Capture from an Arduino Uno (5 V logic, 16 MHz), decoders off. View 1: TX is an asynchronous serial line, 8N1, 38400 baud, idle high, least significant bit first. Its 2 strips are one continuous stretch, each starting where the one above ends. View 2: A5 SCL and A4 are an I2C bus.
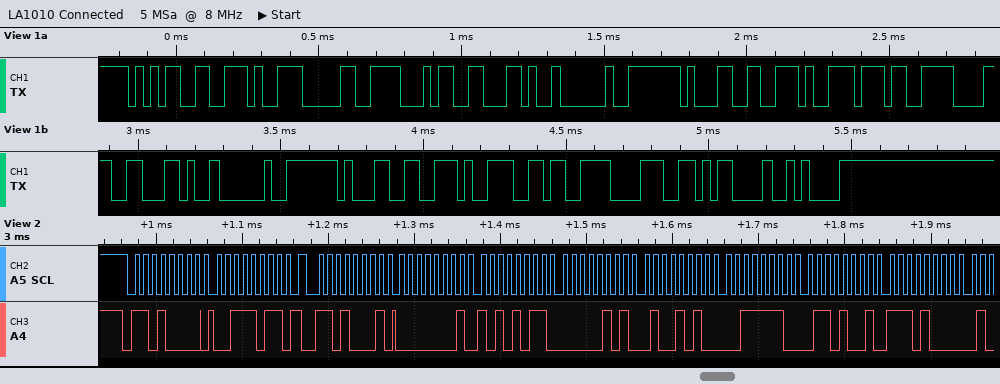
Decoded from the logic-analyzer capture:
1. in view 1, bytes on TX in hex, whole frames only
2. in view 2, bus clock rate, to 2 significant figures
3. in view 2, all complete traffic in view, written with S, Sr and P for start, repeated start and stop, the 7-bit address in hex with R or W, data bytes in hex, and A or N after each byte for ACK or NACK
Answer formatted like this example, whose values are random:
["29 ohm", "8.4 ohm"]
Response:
["35 2E 30 34 2C 20 31 2E 37 38 2C 20 31 2E 36 38 0D 0A", "100 kHz", "S 68W A 3B A Sr 68R A 01 A AB A 05 A 4A A 3E A 69 A E8 A"]
